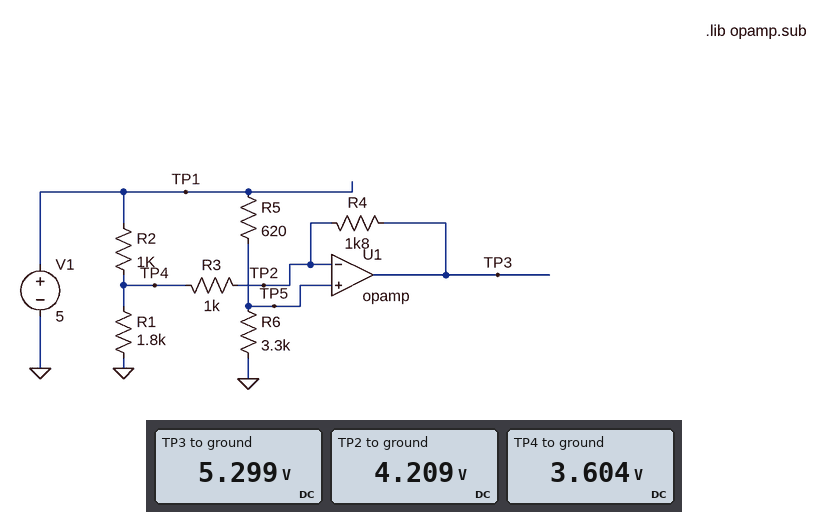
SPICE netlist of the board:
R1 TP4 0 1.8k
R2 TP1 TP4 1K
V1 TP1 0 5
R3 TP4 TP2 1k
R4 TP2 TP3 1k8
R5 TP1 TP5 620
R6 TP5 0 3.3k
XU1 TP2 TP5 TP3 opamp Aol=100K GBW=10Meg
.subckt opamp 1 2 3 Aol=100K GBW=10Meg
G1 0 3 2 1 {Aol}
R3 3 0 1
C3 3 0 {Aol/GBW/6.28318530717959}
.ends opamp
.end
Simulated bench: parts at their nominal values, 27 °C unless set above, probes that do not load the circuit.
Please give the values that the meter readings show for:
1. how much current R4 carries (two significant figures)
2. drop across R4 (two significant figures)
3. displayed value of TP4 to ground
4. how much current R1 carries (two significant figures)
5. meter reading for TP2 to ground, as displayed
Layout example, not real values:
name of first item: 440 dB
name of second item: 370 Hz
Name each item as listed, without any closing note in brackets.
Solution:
how much current R4 carries: 610 µA
drop across R4: 1.1 V
displayed value of TP4 to ground: 3.604 V
how much current R1 carries: 2.0 mA
meter reading for TP2 to ground, as displayed: 4.209 V
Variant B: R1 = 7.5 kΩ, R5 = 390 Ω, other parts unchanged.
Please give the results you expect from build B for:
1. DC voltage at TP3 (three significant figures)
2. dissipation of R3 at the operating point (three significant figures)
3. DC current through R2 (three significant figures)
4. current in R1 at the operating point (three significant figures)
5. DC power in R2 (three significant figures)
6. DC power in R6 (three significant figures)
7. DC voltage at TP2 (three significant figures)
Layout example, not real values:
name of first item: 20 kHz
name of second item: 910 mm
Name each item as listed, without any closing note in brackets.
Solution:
DC voltage at TP3: 4.53 V
dissipation of R3 at the operating point: 1.01 µW
DC current through R2: 560 µA
current in R1 at the operating point: 592 µA
DC power in R2: 314 µW
DC power in R6: 6.06 mW
DC voltage at TP2: 4.47 V
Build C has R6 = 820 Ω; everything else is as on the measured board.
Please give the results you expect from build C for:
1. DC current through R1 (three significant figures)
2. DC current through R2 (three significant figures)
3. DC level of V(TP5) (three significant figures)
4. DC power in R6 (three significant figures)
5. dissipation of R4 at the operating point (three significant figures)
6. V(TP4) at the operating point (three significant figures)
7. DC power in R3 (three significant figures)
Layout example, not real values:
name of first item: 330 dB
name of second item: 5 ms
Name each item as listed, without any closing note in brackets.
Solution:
DC current through R1: 1.71 mA
DC current through R2: 1.93 mA
DC level of V(TP5): 2.85 V
DC power in R6: 9.89 mW
dissipation of R4 at the operating point: 89.9 µW
V(TP4) at the operating point: 3.07 V
DC power in R3: 49.9 µW
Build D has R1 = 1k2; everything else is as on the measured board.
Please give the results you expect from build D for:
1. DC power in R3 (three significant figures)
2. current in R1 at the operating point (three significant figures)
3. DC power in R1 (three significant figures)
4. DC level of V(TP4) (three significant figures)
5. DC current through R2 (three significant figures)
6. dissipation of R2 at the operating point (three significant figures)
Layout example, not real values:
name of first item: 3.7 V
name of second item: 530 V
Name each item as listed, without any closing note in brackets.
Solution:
DC power in R3: 919 µW
current in R1 at the operating point: 2.71 mA
DC power in R1: 8.80 mW
DC level of V(TP4): 3.25 V
DC current through R2: 1.75 mA
dissipation of R2 at the operating point: 3.06 mW
